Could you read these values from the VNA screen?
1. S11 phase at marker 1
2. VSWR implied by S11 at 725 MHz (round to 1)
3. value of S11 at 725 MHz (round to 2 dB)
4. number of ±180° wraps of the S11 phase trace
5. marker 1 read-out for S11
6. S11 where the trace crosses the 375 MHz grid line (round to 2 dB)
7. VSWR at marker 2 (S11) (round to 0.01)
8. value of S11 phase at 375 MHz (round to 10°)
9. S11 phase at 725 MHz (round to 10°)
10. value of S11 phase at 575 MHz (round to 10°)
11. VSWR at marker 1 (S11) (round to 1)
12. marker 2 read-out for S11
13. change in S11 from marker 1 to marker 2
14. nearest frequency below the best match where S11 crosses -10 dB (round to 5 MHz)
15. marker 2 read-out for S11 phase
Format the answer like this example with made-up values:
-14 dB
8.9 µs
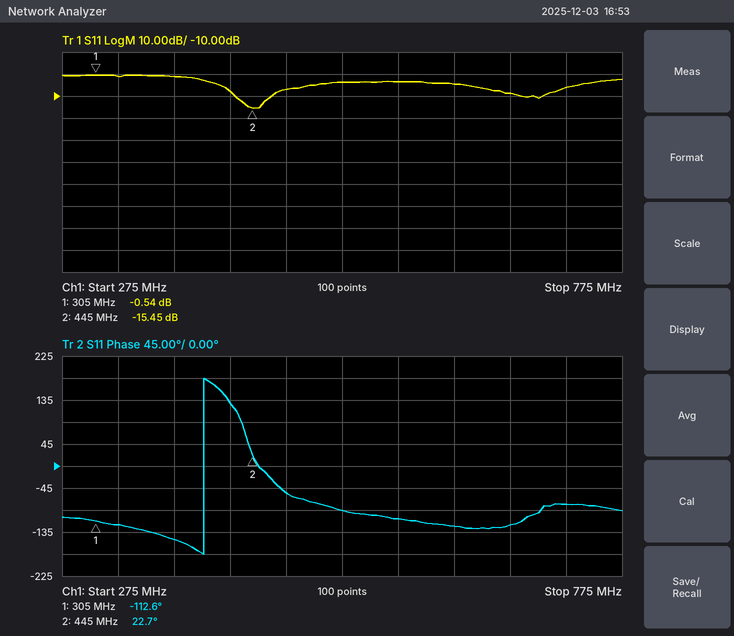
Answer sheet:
-112.6°
3
-6 dB
1
-0.54 dB
-2 dB
1.41
-150°
-80°
-110°
32
-15.45 dB
-14.91 dB
430 MHz
22.7°
